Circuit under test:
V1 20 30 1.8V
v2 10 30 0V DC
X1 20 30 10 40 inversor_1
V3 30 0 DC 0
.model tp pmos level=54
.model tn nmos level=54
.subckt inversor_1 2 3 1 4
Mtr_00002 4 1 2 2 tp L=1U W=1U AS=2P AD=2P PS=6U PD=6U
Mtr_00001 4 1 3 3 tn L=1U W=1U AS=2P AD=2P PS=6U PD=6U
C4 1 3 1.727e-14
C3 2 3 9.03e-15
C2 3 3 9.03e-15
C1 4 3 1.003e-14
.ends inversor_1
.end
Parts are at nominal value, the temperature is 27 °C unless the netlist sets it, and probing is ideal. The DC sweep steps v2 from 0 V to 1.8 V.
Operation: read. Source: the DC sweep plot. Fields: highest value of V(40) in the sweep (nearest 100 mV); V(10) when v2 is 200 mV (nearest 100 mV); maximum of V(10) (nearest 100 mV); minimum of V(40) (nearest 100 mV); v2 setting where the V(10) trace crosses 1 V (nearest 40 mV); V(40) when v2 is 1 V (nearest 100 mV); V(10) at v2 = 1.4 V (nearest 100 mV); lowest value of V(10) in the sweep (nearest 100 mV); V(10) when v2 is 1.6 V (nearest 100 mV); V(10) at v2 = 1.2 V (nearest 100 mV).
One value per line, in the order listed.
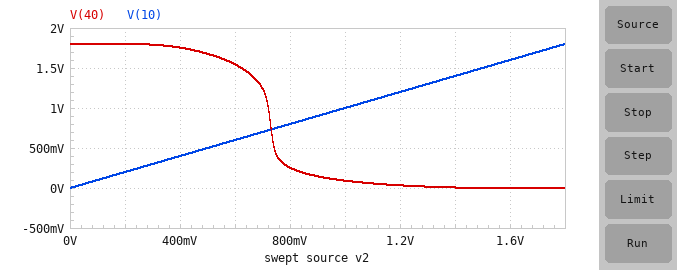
1.8 V
200 mV
1.8 V
0 V
1.00 V
100 mV
1.4 V
0 V
1.6 V
1.2 V
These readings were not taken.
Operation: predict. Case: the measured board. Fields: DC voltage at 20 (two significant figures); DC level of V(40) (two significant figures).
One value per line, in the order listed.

1.8 V
1.8 V
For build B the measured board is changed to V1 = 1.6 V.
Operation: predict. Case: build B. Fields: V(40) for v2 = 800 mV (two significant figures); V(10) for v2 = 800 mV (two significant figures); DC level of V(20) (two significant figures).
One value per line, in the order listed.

130 mV
800 mV
1.6 V
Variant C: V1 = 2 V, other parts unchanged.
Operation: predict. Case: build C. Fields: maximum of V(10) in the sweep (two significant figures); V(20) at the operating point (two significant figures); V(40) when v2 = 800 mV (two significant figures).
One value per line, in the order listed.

1.8 V
2.0 V
960 mV
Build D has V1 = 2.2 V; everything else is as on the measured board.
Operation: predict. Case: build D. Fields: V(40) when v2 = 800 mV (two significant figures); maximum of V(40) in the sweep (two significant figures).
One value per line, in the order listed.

1.7 V
2.2 V
